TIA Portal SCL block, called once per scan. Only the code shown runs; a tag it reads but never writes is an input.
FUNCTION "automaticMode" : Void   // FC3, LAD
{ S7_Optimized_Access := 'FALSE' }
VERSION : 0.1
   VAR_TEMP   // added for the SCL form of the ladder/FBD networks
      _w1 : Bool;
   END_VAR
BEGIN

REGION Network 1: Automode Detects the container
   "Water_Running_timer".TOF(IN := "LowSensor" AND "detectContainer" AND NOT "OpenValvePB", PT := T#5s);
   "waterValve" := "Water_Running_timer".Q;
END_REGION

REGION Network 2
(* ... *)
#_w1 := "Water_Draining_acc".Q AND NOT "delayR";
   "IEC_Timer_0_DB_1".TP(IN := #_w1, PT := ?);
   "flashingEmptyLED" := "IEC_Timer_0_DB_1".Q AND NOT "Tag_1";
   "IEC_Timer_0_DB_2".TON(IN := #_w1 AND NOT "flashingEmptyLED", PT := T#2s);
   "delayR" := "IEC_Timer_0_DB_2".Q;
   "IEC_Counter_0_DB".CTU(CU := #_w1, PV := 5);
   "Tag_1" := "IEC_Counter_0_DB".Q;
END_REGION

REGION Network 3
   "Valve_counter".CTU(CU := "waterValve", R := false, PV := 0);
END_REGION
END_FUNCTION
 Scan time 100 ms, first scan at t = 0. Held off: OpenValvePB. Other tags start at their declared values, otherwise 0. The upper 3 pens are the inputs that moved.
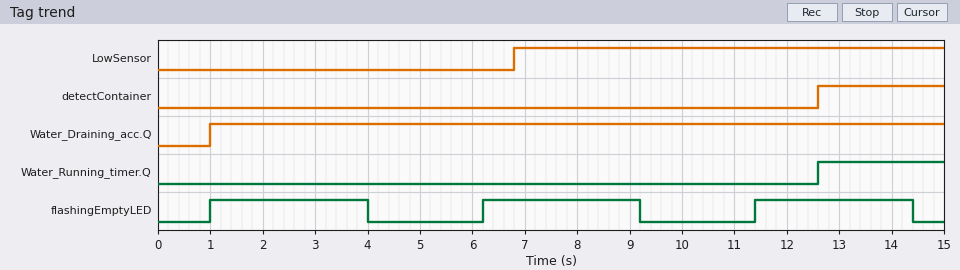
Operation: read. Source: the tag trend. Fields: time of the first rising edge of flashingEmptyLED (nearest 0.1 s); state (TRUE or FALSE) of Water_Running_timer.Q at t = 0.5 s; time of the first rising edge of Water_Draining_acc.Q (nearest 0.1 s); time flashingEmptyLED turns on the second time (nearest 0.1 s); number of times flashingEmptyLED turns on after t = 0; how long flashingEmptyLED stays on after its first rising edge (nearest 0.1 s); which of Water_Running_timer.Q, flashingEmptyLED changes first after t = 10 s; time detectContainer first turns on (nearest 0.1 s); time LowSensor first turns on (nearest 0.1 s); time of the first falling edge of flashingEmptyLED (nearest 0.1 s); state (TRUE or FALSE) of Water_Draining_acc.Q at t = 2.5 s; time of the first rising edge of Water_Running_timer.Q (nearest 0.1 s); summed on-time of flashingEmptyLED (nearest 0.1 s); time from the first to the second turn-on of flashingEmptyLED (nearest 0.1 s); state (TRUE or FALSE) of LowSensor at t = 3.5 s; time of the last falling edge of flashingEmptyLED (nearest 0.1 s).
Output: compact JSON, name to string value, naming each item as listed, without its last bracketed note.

{"time of the first rising edge of flashingEmptyLED": "1.0 s", "state (TRUE or FALSE) of Water_Running_timer.Q at t = 0.5 s": "FALSE", "time of the first rising edge of Water_Draining_acc.Q": "1.0 s", "time flashingEmptyLED turns on the second time": "6.2 s", "number of times flashingEmptyLED turns on after t = 0": "3", "how long flashingEmptyLED stays on after its first rising edge": "3.0 s", "which of Water_Running_timer.Q, flashingEmptyLED changes first after t = 10 s": "flashingEmptyLED", "time detectContainer first turns on": "12.6 s", "time LowSensor first turns on": "6.8 s", "time of the first falling edge of flashingEmptyLED": "4.0 s", "state (TRUE or FALSE) of Water_Draining_acc.Q at t = 2.5 s": "TRUE", "time of the first rising edge of Water_Running_timer.Q": "12.6 s", "summed on-time of flashingEmptyLED": "9.0 s", "time from the first to the second turn-on of flashingEmptyLED": "5.2 s", "state (TRUE or FALSE) of LowSensor at t = 3.5 s": "FALSE", "time of the last falling edge of flashingEmptyLED": "14.4 s"}
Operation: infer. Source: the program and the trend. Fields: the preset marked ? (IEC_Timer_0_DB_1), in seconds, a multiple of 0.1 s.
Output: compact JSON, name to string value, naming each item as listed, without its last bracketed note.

{"the preset marked ? (IEC_Timer_0_DB_1), in seconds, a multiple of 0.1 s": "3.0 s"}
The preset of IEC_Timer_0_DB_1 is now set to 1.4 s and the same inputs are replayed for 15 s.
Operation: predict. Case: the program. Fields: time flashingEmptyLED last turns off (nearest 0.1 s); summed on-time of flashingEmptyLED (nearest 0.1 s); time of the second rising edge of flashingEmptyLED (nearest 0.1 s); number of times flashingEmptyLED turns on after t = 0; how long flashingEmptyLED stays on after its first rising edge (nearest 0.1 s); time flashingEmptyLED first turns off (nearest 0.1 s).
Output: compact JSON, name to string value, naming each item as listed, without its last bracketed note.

{"time flashingEmptyLED last turns off": "13.2 s", "summed on-time of flashingEmptyLED": "5.6 s", "time of the second rising edge of flashingEmptyLED": "4.6 s", "number of times flashingEmptyLED turns on after t = 0": "4", "how long flashingEmptyLED stays on after its first rising edge": "1.4 s", "time flashingEmptyLED first turns off": "2.4 s"}
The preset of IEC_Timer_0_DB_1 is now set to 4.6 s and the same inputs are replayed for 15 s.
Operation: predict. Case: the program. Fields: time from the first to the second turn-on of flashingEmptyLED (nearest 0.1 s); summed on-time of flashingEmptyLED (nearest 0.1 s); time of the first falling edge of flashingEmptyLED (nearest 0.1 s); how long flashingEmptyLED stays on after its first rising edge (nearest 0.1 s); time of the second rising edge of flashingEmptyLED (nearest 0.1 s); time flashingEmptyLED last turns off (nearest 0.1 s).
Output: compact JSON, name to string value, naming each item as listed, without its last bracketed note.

{"time from the first to the second turn-on of flashingEmptyLED": "6.8 s", "summed on-time of flashingEmptyLED": "9.6 s", "time of the first falling edge of flashingEmptyLED": "5.6 s", "how long flashingEmptyLED stays on after its first rising edge": "4.6 s", "time of the second rising edge of flashingEmptyLED": "7.8 s", "time flashingEmptyLED last turns off": "12.4 s"}
